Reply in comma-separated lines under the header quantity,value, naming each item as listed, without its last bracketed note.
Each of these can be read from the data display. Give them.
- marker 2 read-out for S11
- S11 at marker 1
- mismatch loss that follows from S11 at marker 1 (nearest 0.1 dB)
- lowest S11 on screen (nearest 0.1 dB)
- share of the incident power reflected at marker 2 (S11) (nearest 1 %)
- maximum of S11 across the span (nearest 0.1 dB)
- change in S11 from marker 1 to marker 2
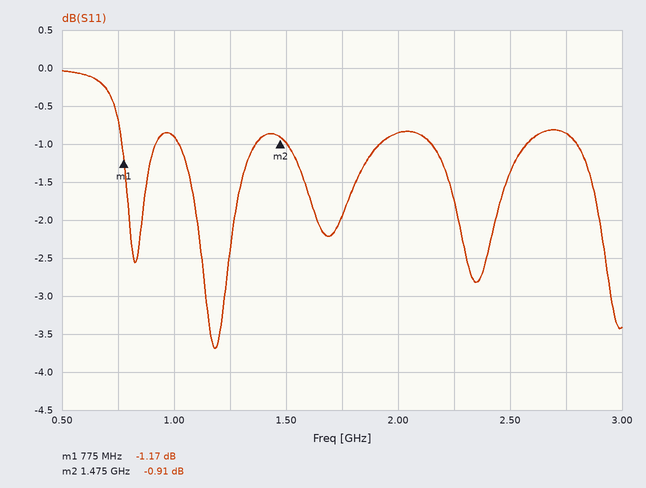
quantity,value
marker 2 read-out for S11,-0.91 dB
S11 at marker 1,-1.17 dB
mismatch loss that follows from S11 at marker 1,6.3 dB
lowest S11 on screen,-3.7 dB
share of the incident power reflected at marker 2 (S11),81 %
maximum of S11 across the span,0.0 dB
change in S11 from marker 1 to marker 2,0.26 dB
